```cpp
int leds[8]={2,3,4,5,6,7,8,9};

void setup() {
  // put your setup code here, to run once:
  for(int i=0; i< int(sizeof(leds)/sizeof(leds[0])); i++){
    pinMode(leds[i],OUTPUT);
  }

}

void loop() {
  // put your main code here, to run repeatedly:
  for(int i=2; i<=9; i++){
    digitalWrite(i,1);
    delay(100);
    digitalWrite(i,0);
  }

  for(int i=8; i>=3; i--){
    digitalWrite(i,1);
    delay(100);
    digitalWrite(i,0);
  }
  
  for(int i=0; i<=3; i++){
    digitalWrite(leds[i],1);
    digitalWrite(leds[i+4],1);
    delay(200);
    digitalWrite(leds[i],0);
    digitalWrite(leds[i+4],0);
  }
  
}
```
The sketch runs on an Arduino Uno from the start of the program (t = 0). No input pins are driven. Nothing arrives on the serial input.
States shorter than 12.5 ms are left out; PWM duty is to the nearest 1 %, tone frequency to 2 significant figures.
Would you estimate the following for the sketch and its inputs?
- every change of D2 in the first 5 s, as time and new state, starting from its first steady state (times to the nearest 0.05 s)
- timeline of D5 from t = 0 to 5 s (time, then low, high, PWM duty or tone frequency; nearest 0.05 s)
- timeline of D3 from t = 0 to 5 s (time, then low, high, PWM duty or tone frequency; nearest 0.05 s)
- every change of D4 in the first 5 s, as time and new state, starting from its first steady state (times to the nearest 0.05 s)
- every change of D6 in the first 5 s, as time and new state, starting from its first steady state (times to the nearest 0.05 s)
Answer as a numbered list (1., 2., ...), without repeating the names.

1. 0 s high; 0.1 s low; 1.4 s high; 1.6 s low; 2.2 s high; 2.3 s low; 3.6 s high; 3.8 s low; 4.4 s high; 4.5 s low
2. 0 s low; 0.3 s high; 0.4 s low; 1.1 s high; 1.2 s low; 2 s high; 2.2 s low; 2.5 s high; 2.6 s low; 3.3 s high; 3.4 s low; 4.2 s high; 4.4 s low; 4.7 s high; 4.8 s low
3. 0 s low; 0.1 s high; 0.2 s low; 1.3 s high; 1.4 s low; 1.6 s high; 1.8 s low; 2.3 s high; 2.4 s low; 3.5 s high; 3.6 s low; 3.8 s high; 4 s low; 4.5 s high; 4.6 s low
4. 0 s low; 0.2 s high; 0.3 s low; 1.2 s high; 1.3 s low; 1.8 s high; 2 s low; 2.4 s high; 2.5 s low; 3.4 s high; 3.5 s low; 4 s high; 4.2 s low; 4.6 s high; 4.7 s low
5. 0 s low; 0.4 s high; 0.5 s low; 1 s high; 1.1 s low; 1.4 s high; 1.6 s low; 2.6 s high; 2.7 s low; 3.2 s high; 3.3 s low; 3.6 s high; 3.8 s low; 4.8 s high; 4.9 s low
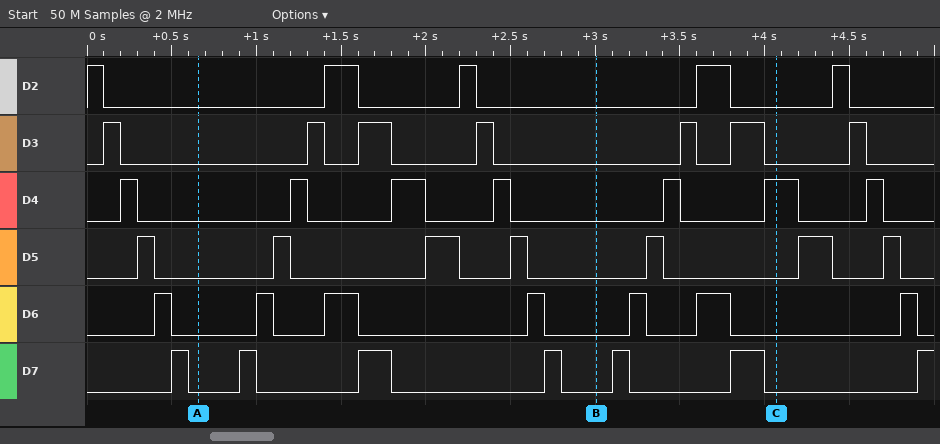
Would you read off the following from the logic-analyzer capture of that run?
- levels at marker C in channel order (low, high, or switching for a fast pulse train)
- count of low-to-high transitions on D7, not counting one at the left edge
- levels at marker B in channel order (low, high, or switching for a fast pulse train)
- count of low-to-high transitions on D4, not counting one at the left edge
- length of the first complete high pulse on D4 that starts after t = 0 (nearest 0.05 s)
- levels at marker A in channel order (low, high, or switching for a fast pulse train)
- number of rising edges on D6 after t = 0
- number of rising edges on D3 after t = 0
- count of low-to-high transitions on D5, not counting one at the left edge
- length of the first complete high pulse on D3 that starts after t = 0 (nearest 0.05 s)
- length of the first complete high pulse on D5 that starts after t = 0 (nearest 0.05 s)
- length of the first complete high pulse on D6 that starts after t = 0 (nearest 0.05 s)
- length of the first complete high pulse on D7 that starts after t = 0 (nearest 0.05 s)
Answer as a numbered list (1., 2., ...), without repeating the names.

1. D2 low, D3 low, D4 high, D5 low, D6 low, D7 low
2. 7
3. D2 low, D3 low, D4 low, D5 low, D6 low, D7 low
4. 7
5. 0.10 s
6. D2 low, D3 low, D4 low, D5 low, D6 low, D7 low
7. 7
8. 7
9. 7
10. 0.10 s
11. 0.10 s
12. 0.10 s
13. 0.10 s
